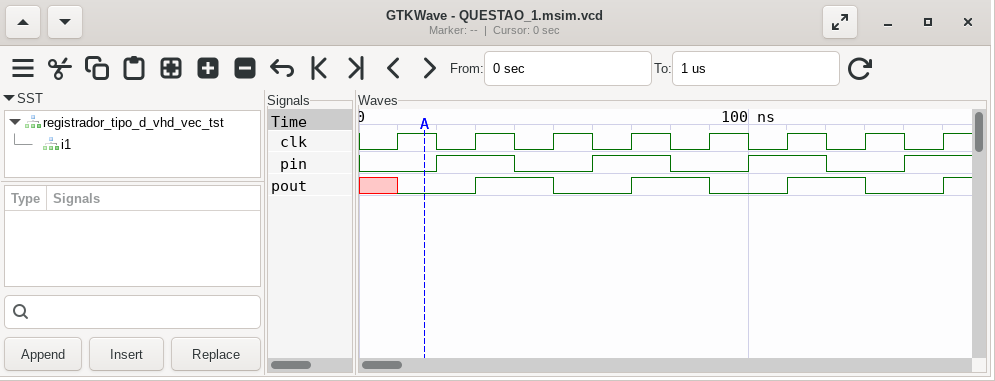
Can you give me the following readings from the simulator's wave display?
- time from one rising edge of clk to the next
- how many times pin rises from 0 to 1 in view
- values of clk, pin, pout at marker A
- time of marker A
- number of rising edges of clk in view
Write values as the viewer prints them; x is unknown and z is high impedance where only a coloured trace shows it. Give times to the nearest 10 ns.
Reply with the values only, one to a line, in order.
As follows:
20 ns
4
clk=1, pin=0, pout=0
20 ns
8
